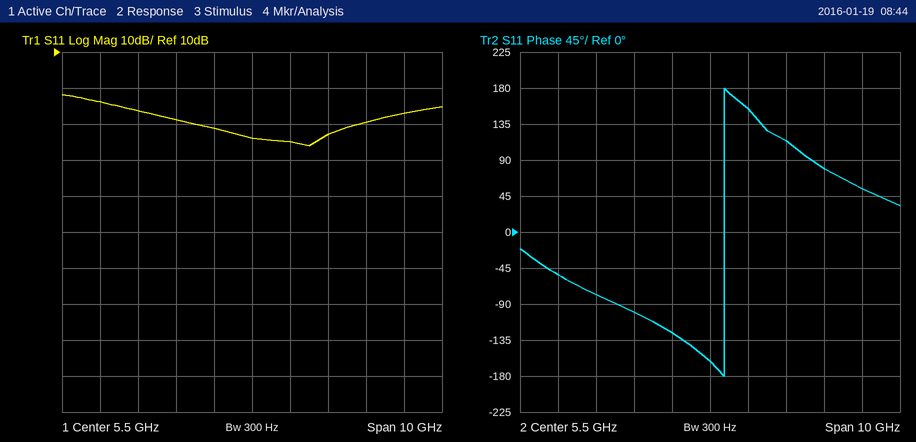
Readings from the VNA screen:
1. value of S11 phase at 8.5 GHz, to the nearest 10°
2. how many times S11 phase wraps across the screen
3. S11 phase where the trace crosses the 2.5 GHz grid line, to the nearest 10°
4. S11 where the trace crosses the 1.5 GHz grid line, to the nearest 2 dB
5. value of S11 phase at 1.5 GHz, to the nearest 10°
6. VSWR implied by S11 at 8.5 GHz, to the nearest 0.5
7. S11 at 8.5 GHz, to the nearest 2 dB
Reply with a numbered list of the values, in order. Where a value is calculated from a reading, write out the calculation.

1. 80°
2. 1
3. -80°
4. -4 dB
5. -50°
6. |Γ| = 10^(-10/20) = 0.3162; VSWR = (1 + 0.3162)/(1 − 0.3162) ≈ 1.92, so 2.0 to the nearest 0.5
7. -10 dB
